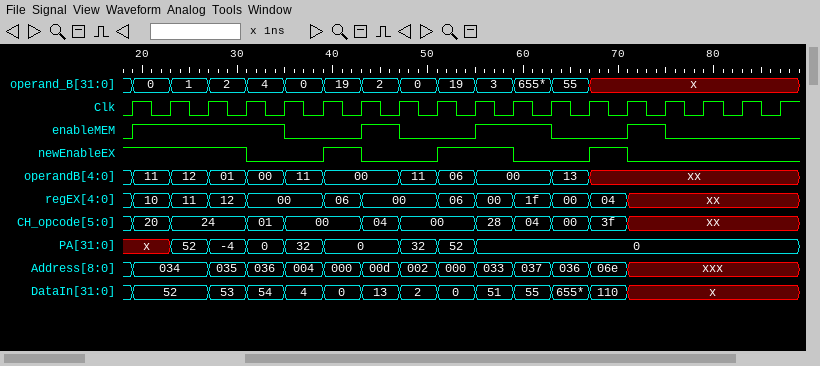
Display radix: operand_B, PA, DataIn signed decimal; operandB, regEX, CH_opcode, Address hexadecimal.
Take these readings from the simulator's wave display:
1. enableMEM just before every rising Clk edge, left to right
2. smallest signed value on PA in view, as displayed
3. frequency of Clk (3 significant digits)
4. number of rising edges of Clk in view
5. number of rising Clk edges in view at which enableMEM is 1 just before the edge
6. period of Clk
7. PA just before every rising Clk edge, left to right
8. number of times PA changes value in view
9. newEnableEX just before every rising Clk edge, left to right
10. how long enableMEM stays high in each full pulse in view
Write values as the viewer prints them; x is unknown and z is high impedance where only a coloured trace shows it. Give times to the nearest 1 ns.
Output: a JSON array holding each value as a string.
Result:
["0 1 1 1 1 0 0 1 0 0 1 1 0 0 1 0 0 0", "-4", "250 MHz", "18", "8", "4 ns", "x, x, 52, -4, 0, 32, 0, 0, 32, 52, 0, 0, 0, 0, 0, 0, 0, 0", "8", "1 1 1 1 0 0 1 0 0 1 1 0 0 1 0 0 0 0", "16 ns, 4 ns, 8 ns, 4 ns"]
